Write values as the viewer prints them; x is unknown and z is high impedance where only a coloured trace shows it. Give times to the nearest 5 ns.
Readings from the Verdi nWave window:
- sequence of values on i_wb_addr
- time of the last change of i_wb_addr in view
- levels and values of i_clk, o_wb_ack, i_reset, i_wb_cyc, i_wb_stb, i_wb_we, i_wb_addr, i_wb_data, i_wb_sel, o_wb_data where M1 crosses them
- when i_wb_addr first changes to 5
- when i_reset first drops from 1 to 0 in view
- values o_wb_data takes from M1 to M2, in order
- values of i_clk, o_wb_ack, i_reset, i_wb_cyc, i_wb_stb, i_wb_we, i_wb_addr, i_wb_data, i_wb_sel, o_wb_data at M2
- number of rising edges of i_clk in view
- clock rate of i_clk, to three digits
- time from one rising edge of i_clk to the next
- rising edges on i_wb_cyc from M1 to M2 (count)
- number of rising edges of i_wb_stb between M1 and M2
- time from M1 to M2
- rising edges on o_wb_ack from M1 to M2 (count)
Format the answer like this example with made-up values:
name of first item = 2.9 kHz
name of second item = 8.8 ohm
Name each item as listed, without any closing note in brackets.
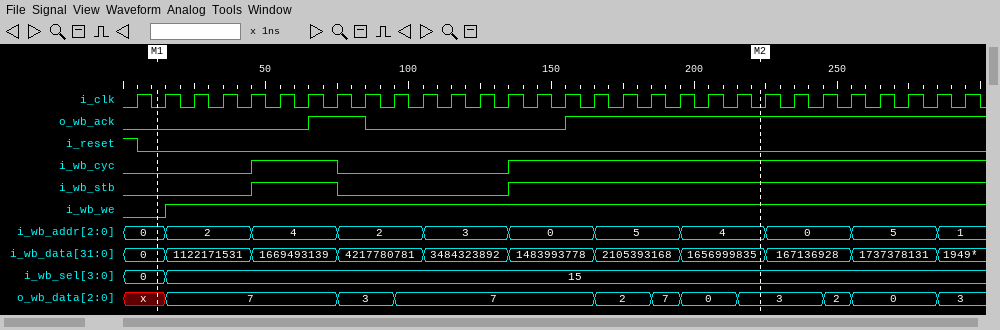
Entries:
sequence of values on i_wb_addr = 0, 2, 4, 2, 3, 0, 5, 4, 0, 5, 1
time of the last change of i_wb_addr in view = 285 ns
levels and values of i_clk, o_wb_ack, i_reset, i_wb_cyc, i_wb_stb, i_wb_we, i_wb_addr, i_wb_data, i_wb_sel, o_wb_data where M1 crosses them = i_clk=0, o_wb_ack=0, i_reset=0, i_wb_cyc=0, i_wb_stb=0, i_wb_we=0, i_wb_addr=0, i_wb_data=0, i_wb_sel=0, o_wb_data=x
when i_wb_addr first changes to 5 = 165 ns
when i_reset first drops from 1 to 0 in view = 5 ns
values o_wb_data takes from M1 to M2, in order = x, 7, 3, 7, 2, 7, 0, 3
values of i_clk, o_wb_ack, i_reset, i_wb_cyc, i_wb_stb, i_wb_we, i_wb_addr, i_wb_data, i_wb_sel, o_wb_data at M2 = i_clk=0, o_wb_ack=1, i_reset=0, i_wb_cyc=1, i_wb_stb=1, i_wb_we=1, i_wb_addr=4, i_wb_data=1656999835, i_wb_sel=15, o_wb_data=3
number of rising edges of i_clk in view = 30
clock rate of i_clk, to three digits = 100 MHz
time from one rising edge of i_clk to the next = 10 ns
rising edges on i_wb_cyc from M1 to M2 = 2
number of rising edges of i_wb_stb between M1 and M2 = 2
time from M1 to M2 = 210 ns
rising edges on o_wb_ack from M1 to M2 = 2
